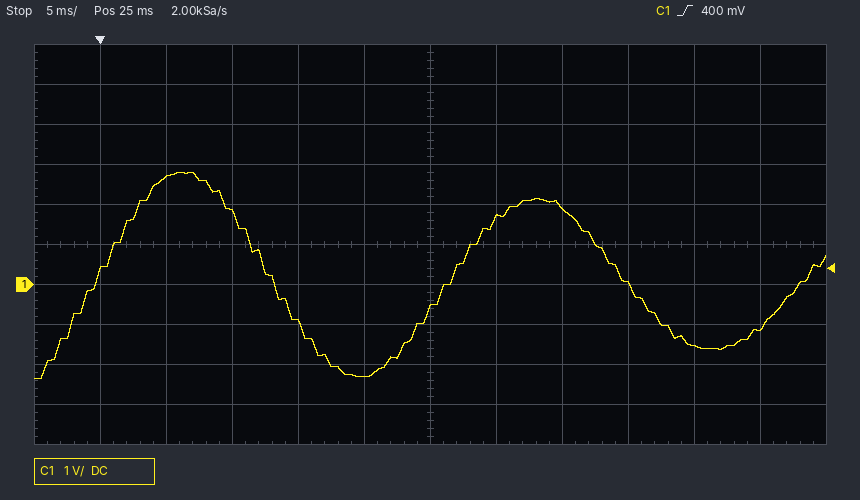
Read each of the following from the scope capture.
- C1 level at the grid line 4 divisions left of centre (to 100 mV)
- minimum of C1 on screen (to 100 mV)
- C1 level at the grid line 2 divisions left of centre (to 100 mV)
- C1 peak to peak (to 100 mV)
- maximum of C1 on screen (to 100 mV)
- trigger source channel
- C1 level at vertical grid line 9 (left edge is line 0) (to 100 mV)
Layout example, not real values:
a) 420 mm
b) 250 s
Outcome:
a) 2.7 V
b) -2.4 V
c) -1.0 V
d) 5.2 V
e) 2.8 V
f) C1
g) 0.0 V
